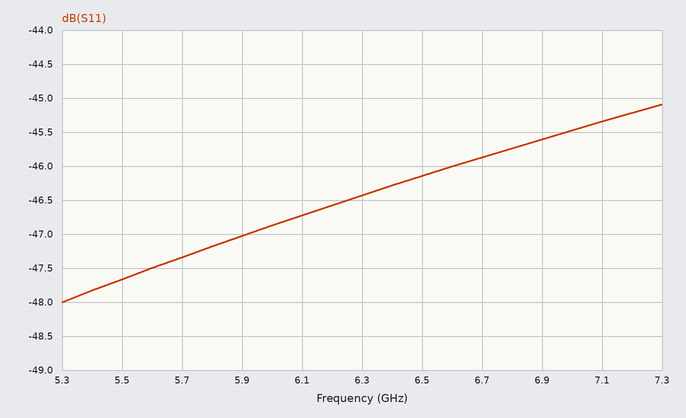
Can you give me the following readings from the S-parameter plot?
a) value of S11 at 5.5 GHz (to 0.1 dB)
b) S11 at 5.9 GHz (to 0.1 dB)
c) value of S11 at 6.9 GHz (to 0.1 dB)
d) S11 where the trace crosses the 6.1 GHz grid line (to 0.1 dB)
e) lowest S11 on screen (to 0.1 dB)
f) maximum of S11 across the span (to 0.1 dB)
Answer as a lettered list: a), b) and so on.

a) -47.7 dB
b) -47.0 dB
c) -45.6 dB
d) -46.7 dB
e) -48.0 dB
f) -45.1 dB
